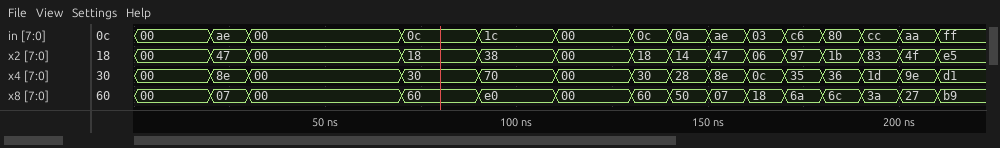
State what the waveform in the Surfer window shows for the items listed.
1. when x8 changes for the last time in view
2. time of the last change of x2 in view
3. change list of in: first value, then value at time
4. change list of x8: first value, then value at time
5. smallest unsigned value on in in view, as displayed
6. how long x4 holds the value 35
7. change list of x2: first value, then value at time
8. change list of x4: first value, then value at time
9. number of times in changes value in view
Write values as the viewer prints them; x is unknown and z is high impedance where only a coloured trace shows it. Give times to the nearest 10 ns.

210 ns
210 ns
00, ae at 20 ns, 00 at 30 ns, 0c at 70 ns, 1c at 90 ns, 00 at 110 ns, 0c at 130 ns, 0a at 140 ns, ae at 150 ns, 03 at 160 ns, c6 at 170 ns, 80 at 180 ns, cc at 190 ns, aa at 200 ns, ff at 210 ns
00, 07 at 20 ns, 00 at 30 ns, 60 at 70 ns, e0 at 90 ns, 00 at 110 ns, 60 at 130 ns, 50 at 140 ns, 07 at 150 ns, 18 at 160 ns, 6a at 170 ns, 6c at 180 ns, 3a at 190 ns, 27 at 200 ns, b9 at 210 ns
00
10 ns
00, 47 at 20 ns, 00 at 30 ns, 18 at 70 ns, 38 at 90 ns, 00 at 110 ns, 18 at 130 ns, 14 at 140 ns, 47 at 150 ns, 06 at 160 ns, 97 at 170 ns, 1b at 180 ns, 83 at 190 ns, 4f at 200 ns, e5 at 210 ns
00, 8e at 20 ns, 00 at 30 ns, 30 at 70 ns, 70 at 90 ns, 00 at 110 ns, 30 at 130 ns, 28 at 140 ns, 8e at 150 ns, 0c at 160 ns, 35 at 170 ns, 36 at 180 ns, 1d at 190 ns, 9e at 200 ns, d1 at 210 ns
14
